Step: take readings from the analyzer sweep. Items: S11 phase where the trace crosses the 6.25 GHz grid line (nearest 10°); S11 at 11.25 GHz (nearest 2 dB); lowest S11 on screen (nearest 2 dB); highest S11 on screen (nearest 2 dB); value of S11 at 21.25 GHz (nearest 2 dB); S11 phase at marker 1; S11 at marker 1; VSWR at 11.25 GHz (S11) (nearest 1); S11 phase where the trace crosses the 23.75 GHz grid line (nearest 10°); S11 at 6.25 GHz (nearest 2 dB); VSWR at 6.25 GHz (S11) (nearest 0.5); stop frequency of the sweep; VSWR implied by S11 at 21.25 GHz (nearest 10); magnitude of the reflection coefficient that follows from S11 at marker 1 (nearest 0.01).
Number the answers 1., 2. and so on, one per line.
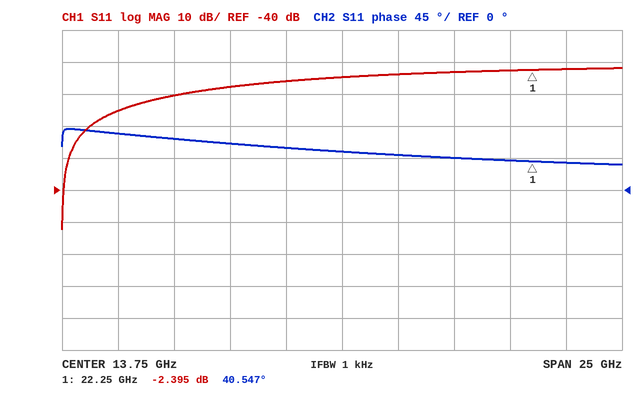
1. 70°
2. -6 dB
3. -52 dB
4. -2 dB
5. -2 dB
6. 40.547°
7. -2.395 dB
8. 3
9. 40°
10. -10 dB
11. 2.0
12. 26.25 GHz
13. 10
14. 0.76
